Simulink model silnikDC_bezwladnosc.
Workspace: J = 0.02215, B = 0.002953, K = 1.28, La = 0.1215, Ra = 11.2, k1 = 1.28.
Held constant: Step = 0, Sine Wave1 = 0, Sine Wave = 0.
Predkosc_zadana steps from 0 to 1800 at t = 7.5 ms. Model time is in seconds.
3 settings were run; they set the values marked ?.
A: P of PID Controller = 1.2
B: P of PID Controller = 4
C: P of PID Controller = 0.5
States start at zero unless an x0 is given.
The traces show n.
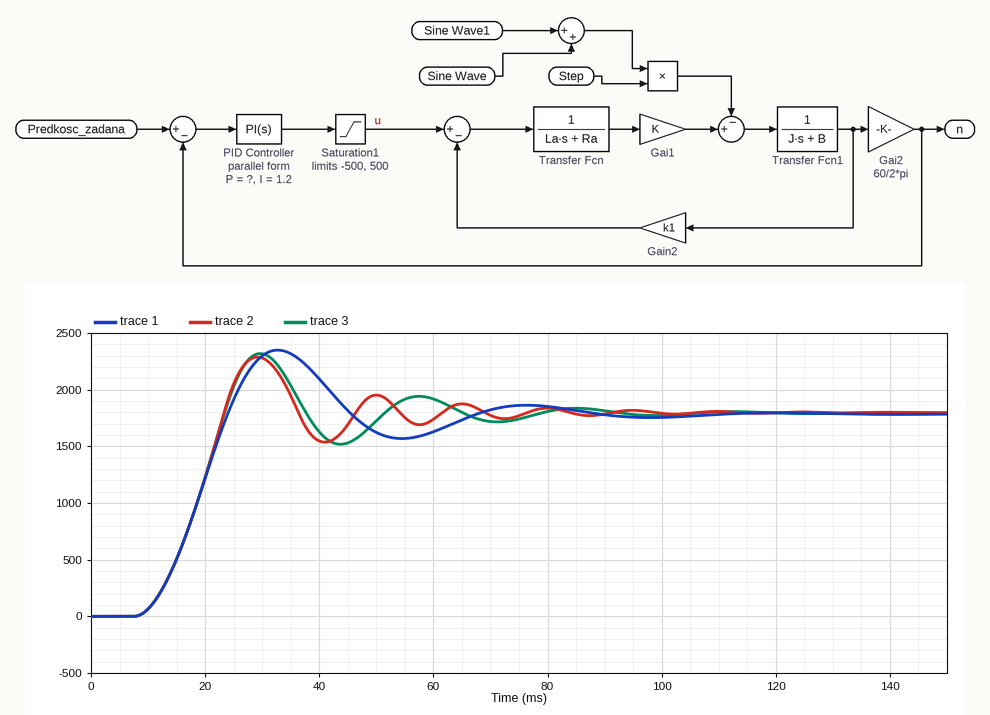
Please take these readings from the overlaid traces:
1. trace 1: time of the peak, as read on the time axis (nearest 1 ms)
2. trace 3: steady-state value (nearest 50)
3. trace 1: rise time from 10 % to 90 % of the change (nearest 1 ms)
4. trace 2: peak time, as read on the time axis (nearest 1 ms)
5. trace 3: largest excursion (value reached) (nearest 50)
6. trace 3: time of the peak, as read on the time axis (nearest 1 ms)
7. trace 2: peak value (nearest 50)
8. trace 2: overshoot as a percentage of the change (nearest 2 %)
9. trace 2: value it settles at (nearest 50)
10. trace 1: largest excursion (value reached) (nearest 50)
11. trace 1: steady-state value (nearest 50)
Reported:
33 ms
1800
11 ms
29 ms
2300
30 ms
2300
28 %
1800
2350
1800
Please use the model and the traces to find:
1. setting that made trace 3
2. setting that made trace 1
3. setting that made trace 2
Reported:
A
C
B
